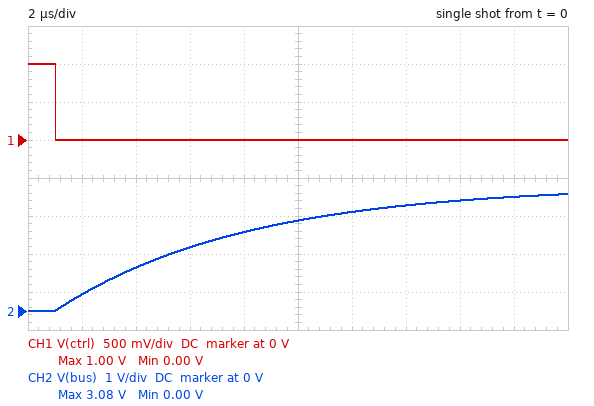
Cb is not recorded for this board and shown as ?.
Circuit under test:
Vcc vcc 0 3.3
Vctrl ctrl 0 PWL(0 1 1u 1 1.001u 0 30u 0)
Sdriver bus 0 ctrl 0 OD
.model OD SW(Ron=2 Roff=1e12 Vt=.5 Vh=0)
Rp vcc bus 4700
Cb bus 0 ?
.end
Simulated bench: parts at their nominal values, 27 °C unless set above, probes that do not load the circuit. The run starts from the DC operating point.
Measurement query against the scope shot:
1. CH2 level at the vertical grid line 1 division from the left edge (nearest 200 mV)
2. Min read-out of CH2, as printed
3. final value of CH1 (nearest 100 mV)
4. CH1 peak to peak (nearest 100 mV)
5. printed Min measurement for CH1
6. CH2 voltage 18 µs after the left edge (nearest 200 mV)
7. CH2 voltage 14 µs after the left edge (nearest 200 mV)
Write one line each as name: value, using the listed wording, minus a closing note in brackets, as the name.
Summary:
CH2 level at the vertical grid line 1 division from the left edge: 400 mV
Min read-out of CH2, as printed: 0.00 V
final value of CH1: 0 V
CH1 peak to peak: 1.0 V
printed Min measurement for CH1: 0.00 V
CH2 voltage 18 µs after the left edge: 3.0 V
CH2 voltage 14 µs after the left edge: 2.8 V
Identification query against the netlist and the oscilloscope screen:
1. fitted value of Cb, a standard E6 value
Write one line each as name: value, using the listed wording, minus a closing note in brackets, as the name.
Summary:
fitted value of Cb, a standard E6 value: 1.5 nF
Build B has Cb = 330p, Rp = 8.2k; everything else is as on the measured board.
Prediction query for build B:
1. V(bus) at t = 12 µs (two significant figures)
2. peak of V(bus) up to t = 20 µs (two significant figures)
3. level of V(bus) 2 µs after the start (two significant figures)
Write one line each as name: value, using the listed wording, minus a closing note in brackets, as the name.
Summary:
V(bus) at t = 12 µs: 3.2 V
peak of V(bus) up to t = 20 µs: 3.3 V
level of V(bus) 2 µs after the start: 1.0 V
